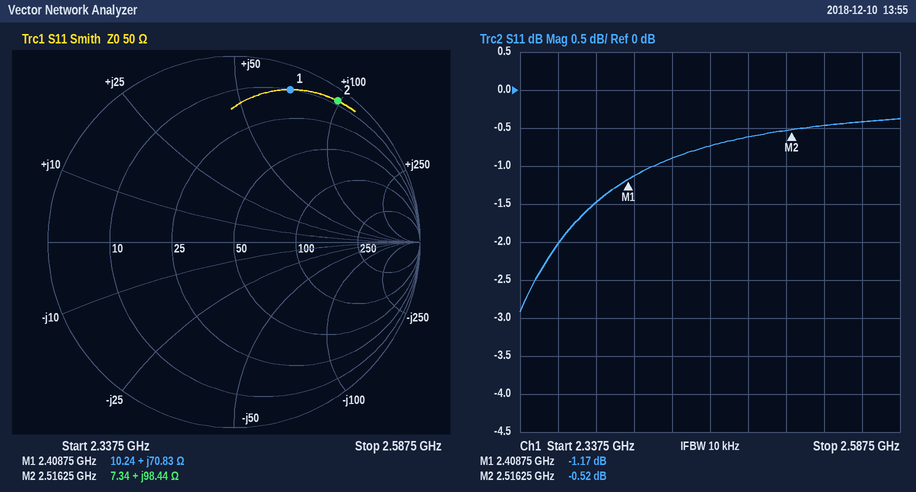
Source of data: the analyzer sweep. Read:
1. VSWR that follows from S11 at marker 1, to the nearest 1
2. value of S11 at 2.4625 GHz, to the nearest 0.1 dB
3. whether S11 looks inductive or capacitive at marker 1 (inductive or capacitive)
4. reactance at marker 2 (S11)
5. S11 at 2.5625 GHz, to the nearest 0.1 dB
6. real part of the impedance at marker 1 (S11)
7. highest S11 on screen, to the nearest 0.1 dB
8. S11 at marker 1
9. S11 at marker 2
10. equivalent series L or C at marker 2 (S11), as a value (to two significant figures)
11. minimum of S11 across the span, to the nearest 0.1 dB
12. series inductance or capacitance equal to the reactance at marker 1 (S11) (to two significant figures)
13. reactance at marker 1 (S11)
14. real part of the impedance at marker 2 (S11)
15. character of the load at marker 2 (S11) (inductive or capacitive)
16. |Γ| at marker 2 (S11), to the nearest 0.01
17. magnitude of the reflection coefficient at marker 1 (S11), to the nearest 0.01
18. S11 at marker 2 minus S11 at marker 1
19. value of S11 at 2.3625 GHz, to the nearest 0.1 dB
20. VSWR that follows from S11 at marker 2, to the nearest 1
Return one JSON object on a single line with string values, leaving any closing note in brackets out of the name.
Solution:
{"VSWR that follows from S11 at marker 1, to the nearest 1": "15", "value of S11 at 2.4625 GHz, to the nearest 0.1 dB": "-0.7 dB", "whether S11 looks inductive or capacitive at marker 1": "inductive", "reactance at marker 2": "+98.44 Ω", "S11 at 2.5625 GHz, to the nearest 0.1 dB": "-0.4 dB", "real part of the impedance at marker 1": "10.24 Ω", "highest S11 on screen, to the nearest 0.1 dB": "-0.4 dB", "S11 at marker 1": "-1.17 dB", "S11 at marker 2": "-0.52 dB", "equivalent series L or C at marker 2 (S11), as a value": "6.2 nH", "minimum of S11 across the span, to the nearest 0.1 dB": "-2.9 dB", "series inductance or capacitance equal to the reactance at marker 1 (S11)": "4.7 nH", "reactance at marker 1": "+70.83 Ω", "real part of the impedance at marker 2": "7.34 Ω", "character of the load at marker 2 (S11)": "inductive", "|Γ| at marker 2 (S11), to the nearest 0.01": "0.94", "magnitude of the reflection coefficient at marker 1 (S11), to the nearest 0.01": "0.87", "S11 at marker 2 minus S11 at marker 1": "0.65 dB", "value of S11 at 2.3625 GHz, to the nearest 0.1 dB": "-2.0 dB", "VSWR that follows from S11 at marker 2, to the nearest 1": "33"}
